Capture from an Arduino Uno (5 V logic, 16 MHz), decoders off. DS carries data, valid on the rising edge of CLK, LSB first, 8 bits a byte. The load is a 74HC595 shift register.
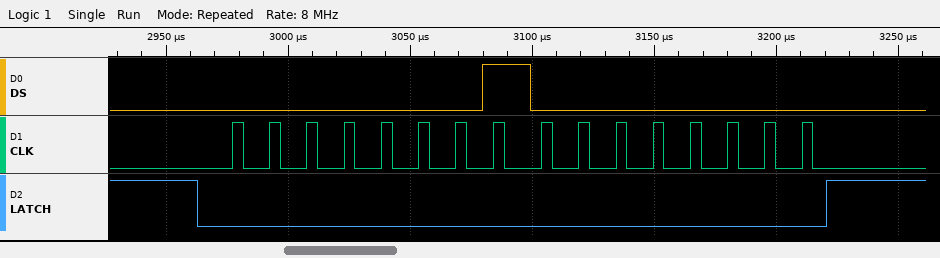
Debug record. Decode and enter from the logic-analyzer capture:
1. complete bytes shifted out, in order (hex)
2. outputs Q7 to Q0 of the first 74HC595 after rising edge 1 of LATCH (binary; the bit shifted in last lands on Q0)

0x80 0x00
00000000
